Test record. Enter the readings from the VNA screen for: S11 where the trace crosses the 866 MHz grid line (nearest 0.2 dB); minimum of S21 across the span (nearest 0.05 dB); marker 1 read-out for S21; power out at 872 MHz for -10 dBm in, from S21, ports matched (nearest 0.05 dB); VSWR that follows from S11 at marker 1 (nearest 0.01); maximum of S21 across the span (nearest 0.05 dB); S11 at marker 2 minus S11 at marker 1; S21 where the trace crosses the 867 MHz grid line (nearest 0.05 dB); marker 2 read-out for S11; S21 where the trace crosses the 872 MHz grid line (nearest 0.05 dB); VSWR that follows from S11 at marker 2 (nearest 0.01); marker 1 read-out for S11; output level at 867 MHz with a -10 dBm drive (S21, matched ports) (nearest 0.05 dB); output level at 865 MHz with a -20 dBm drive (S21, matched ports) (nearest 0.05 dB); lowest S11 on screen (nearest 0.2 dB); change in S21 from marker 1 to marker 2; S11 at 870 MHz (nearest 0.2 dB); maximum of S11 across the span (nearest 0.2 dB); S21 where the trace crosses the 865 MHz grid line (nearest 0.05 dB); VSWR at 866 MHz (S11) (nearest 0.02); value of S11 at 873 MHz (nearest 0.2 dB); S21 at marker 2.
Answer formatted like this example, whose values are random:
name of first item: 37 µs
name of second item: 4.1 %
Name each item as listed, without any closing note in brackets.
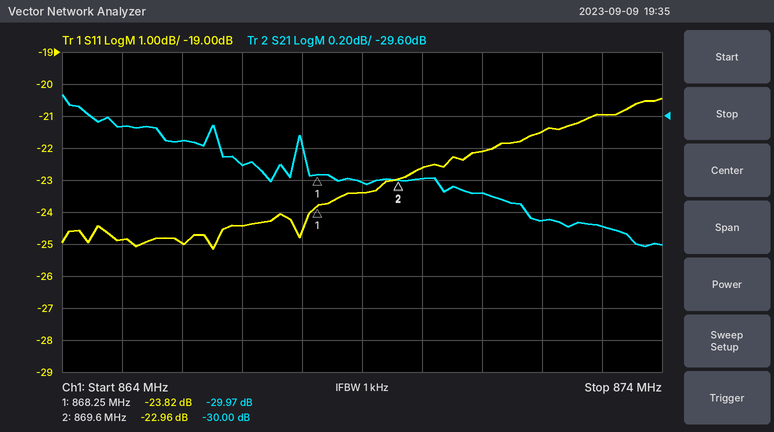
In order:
S11 where the trace crosses the 866 MHz grid line: -25.0 dB
minimum of S21 across the span: -30.40 dB
marker 1 read-out for S21: -29.97 dB
power out at 872 MHz for -10 dBm in, from S21, ports matched: -40.25 dBm
VSWR that follows from S11 at marker 1: 1.14
maximum of S21 across the span: -29.45 dB
S11 at marker 2 minus S11 at marker 1: 0.86 dB
S21 where the trace crosses the 867 MHz grid line: -29.90 dB
marker 2 read-out for S11: -22.96 dB
S21 where the trace crosses the 872 MHz grid line: -30.25 dB
VSWR that follows from S11 at marker 2: 1.15
marker 1 read-out for S11: -23.82 dB
output level at 867 MHz with a -10 dBm drive (S21, matched ports): -39.90 dBm
output level at 865 MHz with a -20 dBm drive (S21, matched ports): -49.65 dBm
lowest S11 on screen: -25.2 dB
change in S21 from marker 1 to marker 2: -0.03 dB
S11 at 870 MHz: -22.6 dB
maximum of S11 across the span: -20.4 dB
S21 where the trace crosses the 865 MHz grid line: -29.65 dB
VSWR at 866 MHz (S11): 1.12
value of S11 at 873 MHz: -21.0 dB
S21 at marker 2: -30.00 dB
